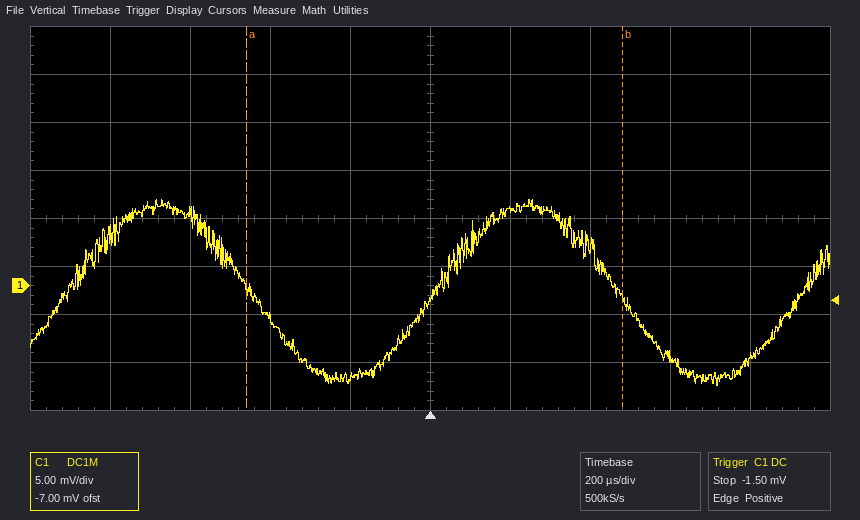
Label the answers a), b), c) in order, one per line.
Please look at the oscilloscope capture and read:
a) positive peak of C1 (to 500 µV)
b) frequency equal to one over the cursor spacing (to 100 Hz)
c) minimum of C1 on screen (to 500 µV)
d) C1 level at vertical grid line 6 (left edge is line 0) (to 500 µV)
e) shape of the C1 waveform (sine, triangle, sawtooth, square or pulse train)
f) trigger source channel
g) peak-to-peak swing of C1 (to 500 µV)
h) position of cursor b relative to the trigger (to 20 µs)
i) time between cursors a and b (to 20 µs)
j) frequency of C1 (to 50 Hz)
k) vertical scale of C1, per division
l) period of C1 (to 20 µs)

a) 9.0 mV
b) 1.1 kHz
c) -10.5 mV
d) 8.0 mV
e) sine
f) C1
g) 19.5 mV
h) +480 µs
i) 940 µs
j) 1.10 kHz
k) 5 mV
l) 920 µs
